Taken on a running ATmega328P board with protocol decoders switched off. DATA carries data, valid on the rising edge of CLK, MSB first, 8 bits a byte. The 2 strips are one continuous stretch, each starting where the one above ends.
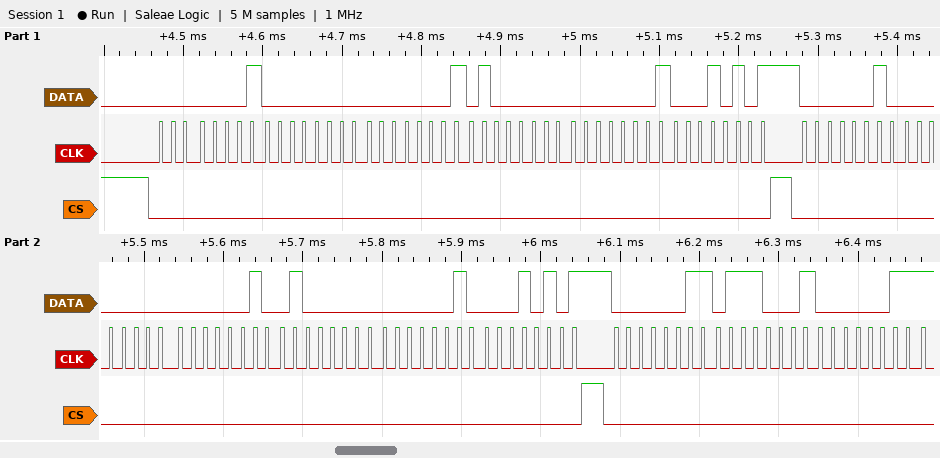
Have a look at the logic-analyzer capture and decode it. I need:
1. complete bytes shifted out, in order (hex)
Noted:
01 00 01 40 01 15 02 00 02 40 02 15 03 71 03
